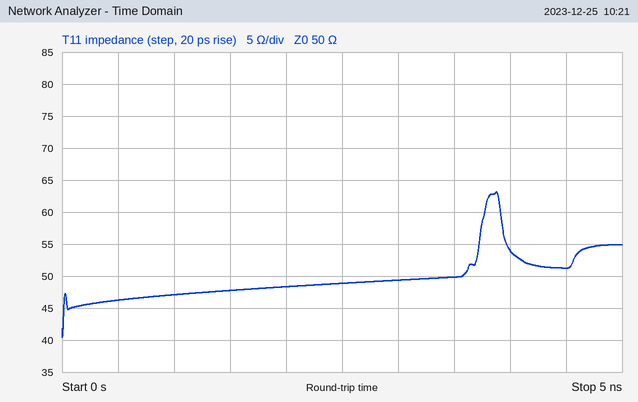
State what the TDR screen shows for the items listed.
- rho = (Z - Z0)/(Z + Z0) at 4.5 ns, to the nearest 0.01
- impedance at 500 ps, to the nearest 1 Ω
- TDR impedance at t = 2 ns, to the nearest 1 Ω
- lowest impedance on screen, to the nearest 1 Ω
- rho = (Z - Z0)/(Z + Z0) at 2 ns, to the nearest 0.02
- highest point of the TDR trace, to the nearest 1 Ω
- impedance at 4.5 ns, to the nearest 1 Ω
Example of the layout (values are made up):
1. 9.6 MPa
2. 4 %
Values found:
1. +0.01
2. 46 Ω
3. 48 Ω
4. 40 Ω
5. -0.02
6. 63 Ω
7. 51 Ω
